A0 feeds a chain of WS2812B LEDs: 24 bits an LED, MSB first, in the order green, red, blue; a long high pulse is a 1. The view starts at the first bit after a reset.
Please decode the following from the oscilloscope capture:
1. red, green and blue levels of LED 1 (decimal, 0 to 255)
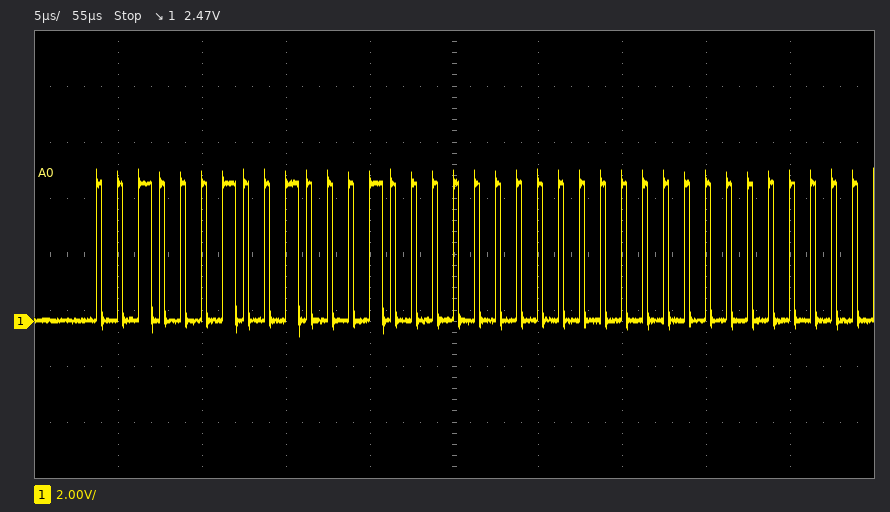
68, 34, 0
